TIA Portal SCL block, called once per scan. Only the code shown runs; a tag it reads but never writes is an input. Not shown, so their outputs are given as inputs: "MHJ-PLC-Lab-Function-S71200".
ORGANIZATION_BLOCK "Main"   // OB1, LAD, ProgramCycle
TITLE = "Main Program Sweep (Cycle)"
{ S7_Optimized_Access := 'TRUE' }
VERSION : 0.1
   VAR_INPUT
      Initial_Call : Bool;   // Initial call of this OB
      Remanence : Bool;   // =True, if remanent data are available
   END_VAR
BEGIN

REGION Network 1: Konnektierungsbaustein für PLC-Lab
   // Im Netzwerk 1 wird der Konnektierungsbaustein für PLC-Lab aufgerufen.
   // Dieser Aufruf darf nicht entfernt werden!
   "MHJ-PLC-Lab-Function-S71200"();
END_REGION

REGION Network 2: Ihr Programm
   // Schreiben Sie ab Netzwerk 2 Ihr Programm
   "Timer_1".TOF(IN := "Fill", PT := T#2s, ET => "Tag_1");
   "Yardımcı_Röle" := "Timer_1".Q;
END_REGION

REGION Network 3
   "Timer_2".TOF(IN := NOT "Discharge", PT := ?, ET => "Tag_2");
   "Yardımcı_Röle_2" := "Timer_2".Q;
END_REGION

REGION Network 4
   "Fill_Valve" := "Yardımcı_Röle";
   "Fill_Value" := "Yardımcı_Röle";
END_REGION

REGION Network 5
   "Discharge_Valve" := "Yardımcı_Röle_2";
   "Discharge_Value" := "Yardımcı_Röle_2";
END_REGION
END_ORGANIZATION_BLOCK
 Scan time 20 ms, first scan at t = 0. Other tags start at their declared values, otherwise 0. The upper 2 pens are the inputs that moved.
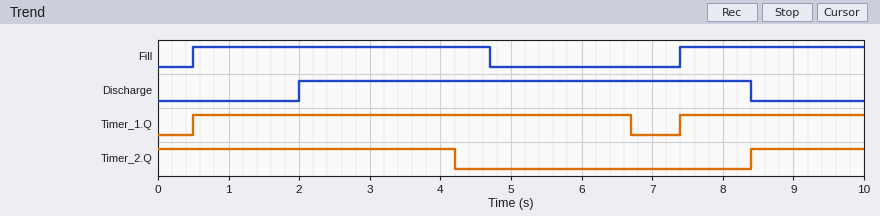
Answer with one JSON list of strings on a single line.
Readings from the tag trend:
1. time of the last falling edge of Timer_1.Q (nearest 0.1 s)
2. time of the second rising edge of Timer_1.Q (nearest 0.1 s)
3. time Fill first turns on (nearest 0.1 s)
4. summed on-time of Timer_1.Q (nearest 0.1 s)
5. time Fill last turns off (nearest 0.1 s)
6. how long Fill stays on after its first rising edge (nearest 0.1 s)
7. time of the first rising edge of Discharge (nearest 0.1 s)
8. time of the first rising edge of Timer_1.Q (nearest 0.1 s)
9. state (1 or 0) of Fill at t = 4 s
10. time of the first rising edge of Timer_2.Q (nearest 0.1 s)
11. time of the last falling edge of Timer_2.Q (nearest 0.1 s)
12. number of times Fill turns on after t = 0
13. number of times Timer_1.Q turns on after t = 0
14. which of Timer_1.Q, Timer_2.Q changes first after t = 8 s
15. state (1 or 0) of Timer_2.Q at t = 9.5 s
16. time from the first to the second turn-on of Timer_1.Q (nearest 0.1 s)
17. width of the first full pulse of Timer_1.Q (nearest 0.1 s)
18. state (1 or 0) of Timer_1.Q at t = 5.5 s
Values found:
["6.7 s", "7.4 s", "0.5 s", "8.8 s", "4.7 s", "4.2 s", "2.0 s", "0.5 s", "1", "8.4 s", "4.2 s", "2", "2", "Timer_2.Q", "1", "6.9 s", "6.2 s", "1"]
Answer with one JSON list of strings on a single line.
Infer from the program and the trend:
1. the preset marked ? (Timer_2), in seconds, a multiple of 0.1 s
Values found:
["2.2 s"]
